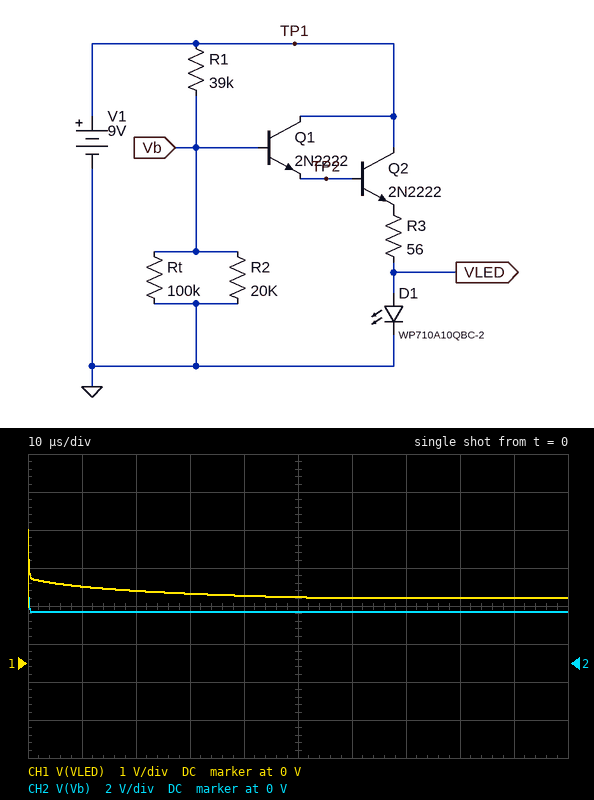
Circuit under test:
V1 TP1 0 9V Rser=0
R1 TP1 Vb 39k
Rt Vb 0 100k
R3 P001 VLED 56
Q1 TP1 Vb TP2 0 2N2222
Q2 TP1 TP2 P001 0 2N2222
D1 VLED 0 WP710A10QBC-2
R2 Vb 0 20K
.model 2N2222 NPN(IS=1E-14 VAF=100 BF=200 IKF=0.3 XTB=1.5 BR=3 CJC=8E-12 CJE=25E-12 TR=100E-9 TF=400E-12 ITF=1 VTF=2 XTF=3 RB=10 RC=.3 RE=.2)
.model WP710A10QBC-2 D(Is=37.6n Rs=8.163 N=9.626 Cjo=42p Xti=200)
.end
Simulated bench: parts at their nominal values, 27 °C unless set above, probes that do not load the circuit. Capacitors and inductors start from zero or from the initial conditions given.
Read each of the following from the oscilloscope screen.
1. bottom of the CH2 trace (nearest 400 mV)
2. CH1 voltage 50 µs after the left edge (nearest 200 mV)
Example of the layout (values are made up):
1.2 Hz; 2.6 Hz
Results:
2.8 V; 1.8 V
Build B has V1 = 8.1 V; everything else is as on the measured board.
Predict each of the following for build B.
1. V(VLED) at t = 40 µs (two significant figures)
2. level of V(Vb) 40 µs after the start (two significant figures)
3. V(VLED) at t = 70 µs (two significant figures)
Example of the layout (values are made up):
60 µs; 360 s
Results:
1.7 V; 2.4 V; 1.6 V
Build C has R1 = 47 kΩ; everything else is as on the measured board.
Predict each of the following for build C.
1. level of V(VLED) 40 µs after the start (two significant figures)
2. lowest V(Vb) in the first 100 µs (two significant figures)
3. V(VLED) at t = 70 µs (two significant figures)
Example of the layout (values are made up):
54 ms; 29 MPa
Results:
1.7 V; 2.3 V; 1.6 V
